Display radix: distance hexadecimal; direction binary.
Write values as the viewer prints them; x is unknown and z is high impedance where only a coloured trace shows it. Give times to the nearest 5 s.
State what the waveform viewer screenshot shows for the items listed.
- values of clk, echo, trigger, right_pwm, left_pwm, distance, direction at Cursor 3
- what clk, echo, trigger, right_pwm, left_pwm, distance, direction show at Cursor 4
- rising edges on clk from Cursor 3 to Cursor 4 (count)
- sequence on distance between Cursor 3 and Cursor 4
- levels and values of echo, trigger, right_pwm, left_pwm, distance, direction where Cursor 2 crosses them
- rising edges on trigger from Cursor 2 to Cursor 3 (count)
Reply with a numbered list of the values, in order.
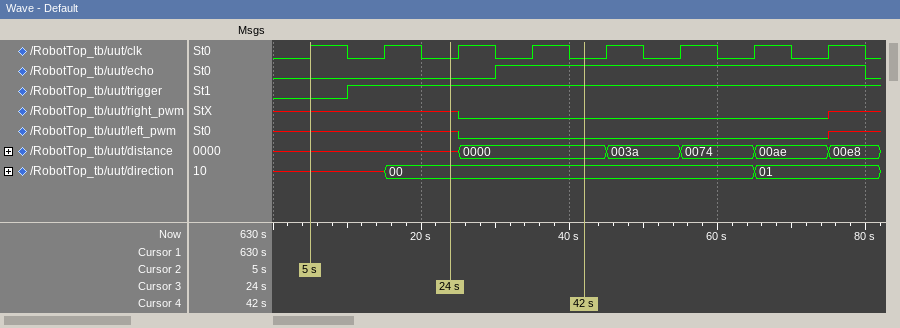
1. clk=0, echo=0, trigger=1, right_pwm=x, left_pwm=x, distance=x, direction=00
2. clk=0, echo=1, trigger=1, right_pwm=0, left_pwm=0, distance=0000, direction=00
3. 2
4. x, 0000
5. echo=0, trigger=0, right_pwm=x, left_pwm=x, distance=x, direction=x
6. 1
